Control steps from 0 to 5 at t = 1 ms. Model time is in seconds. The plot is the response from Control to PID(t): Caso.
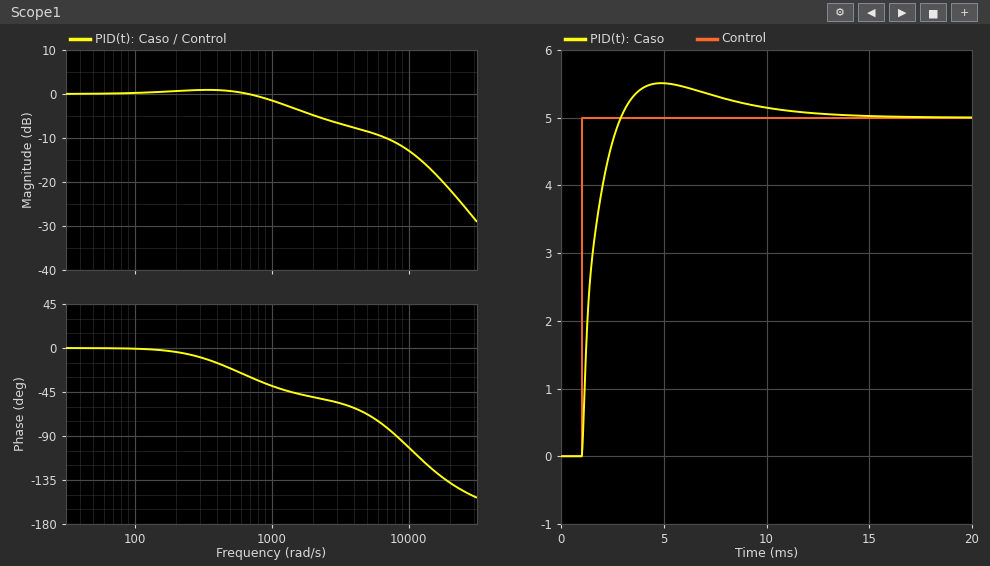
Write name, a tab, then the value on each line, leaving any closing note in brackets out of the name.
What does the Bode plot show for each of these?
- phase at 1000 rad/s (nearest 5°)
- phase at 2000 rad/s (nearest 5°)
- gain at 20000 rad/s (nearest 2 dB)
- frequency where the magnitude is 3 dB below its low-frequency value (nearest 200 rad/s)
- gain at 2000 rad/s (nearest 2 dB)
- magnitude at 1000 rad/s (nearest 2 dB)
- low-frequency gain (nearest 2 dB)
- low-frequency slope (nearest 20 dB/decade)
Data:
phase at 1000 rad/s	-40°
phase at 2000 rad/s	-50°
gain at 20000 rad/s	-22 dB
frequency where the magnitude is 3 dB below its low-frequency value	1400 rad/s
gain at 2000 rad/s	-4 dB
magnitude at 1000 rad/s	-2 dB
low-frequency gain	0 dB
low-frequency slope	0 dB/decade
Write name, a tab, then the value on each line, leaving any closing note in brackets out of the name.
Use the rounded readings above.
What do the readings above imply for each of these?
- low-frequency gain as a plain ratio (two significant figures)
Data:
low-frequency gain as a plain ratio	1.0
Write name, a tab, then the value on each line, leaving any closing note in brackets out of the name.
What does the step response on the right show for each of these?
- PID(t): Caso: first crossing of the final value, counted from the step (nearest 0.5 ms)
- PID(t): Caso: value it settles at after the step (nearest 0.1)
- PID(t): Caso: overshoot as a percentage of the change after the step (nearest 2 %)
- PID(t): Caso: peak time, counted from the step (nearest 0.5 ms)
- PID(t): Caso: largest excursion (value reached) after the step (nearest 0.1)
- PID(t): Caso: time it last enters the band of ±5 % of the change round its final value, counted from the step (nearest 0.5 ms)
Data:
PID(t): Caso: first crossing of the final value, counted from the step	2.0 ms
PID(t): Caso: value it settles at after the step	5.0
PID(t): Caso: overshoot as a percentage of the change after the step	10 %
PID(t): Caso: peak time, counted from the step	4.0 ms
PID(t): Caso: largest excursion (value reached) after the step	5.5
PID(t): Caso: time it last enters the band of ±5 % of the change round its final value, counted from the step	7.5 ms
